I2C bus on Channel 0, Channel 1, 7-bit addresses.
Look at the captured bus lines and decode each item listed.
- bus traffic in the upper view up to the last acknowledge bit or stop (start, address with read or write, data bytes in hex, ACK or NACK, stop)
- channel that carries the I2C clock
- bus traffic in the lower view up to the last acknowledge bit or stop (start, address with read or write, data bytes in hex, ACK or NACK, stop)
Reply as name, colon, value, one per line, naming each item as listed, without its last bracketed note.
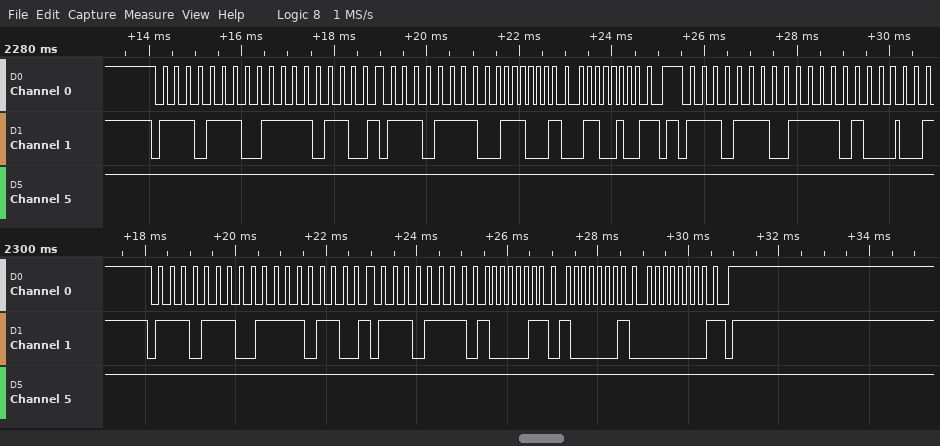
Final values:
bus traffic in the upper view up to the last acknowledge bit or stop: start, address 77 write ACK, F6 ACK, repeated start, address 77 read ACK, 71 ACK, 64 NACK, stop, start, address 77 write ACK, F4 ACK
channel that carries the I2C clock: Channel 0
bus traffic in the lower view up to the last acknowledge bit or stop: start, address 77 write ACK, F6 ACK, repeated start, address 77 read ACK, 83 ACK, 81 ACK, 00 NACK, stop
